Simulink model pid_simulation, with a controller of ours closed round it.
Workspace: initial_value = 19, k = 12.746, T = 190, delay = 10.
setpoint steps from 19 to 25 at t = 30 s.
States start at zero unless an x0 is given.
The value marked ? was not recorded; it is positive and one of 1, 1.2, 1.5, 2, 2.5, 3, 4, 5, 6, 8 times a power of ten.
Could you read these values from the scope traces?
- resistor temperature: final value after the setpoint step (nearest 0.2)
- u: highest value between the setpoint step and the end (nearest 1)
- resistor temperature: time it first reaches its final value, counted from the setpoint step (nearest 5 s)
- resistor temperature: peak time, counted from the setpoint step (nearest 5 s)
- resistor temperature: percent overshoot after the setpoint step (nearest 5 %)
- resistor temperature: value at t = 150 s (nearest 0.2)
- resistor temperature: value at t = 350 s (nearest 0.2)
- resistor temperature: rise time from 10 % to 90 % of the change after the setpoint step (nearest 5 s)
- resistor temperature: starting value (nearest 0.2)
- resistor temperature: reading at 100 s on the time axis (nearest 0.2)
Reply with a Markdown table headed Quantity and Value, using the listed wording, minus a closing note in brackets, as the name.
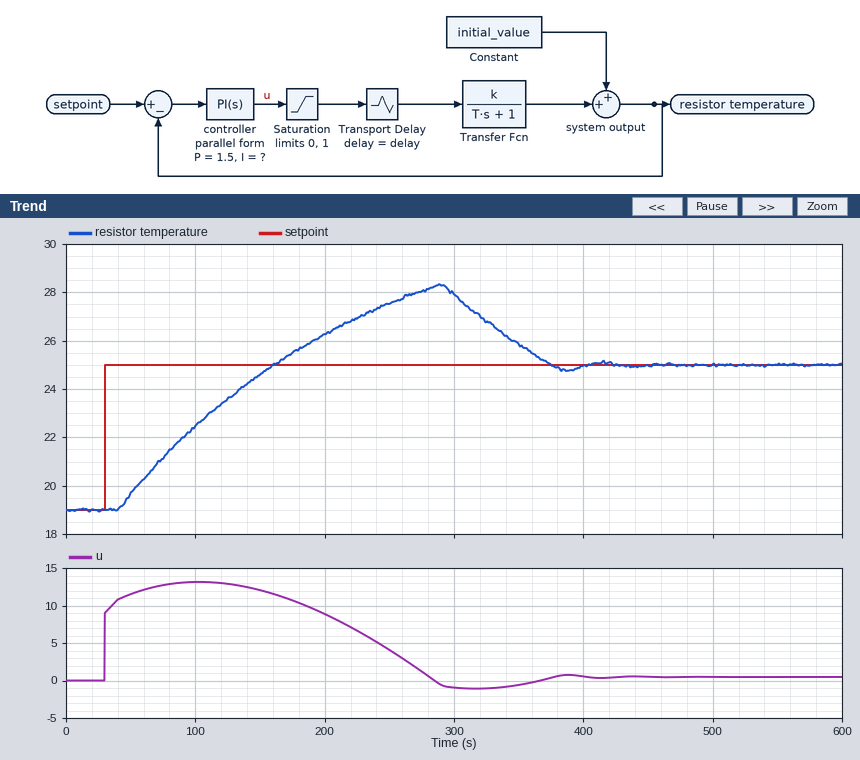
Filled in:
| Quantity | Value |
|---|---|
| resistor temperature: final value after the setpoint step | 25.0 |
| u: highest value between the setpoint step and the end | 13 |
| resistor temperature: time it first reaches its final value, counted from the setpoint step | 130 s |
| resistor temperature: peak time, counted from the setpoint step | 260 s |
| resistor temperature: percent overshoot after the setpoint step | 55 % |
| resistor temperature: value at t = 150 s | 24.6 |
| resistor temperature: value at t = 350 s | 25.8 |
| resistor temperature: rise time from 10 % to 90 % of the change after the setpoint step | 95 s |
| resistor temperature: starting value | 19.0 |
| resistor temperature: reading at 100 s on the time axis | 22.4 |
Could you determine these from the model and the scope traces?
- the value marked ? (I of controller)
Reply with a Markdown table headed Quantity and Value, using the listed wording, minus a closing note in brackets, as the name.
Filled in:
| Quantity | Value |
|---|---|
| the value marked ? | 0.03 |
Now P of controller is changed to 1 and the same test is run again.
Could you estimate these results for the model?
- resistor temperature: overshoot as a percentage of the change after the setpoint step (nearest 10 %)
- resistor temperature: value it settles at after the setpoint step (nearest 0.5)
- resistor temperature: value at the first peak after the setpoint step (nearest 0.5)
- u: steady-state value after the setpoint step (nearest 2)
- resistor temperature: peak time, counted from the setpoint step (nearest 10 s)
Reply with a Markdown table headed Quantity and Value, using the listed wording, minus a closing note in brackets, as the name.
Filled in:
| Quantity | Value |
|---|---|
| resistor temperature: overshoot as a percentage of the change after the setpoint step | 60 % |
| resistor temperature: value it settles at after the setpoint step | 25.0 |
| resistor temperature: value at the first peak after the setpoint step | 28.5 |
| u: steady-state value after the setpoint step | 0 |
| resistor temperature: peak time, counted from the setpoint step | 270 s |
